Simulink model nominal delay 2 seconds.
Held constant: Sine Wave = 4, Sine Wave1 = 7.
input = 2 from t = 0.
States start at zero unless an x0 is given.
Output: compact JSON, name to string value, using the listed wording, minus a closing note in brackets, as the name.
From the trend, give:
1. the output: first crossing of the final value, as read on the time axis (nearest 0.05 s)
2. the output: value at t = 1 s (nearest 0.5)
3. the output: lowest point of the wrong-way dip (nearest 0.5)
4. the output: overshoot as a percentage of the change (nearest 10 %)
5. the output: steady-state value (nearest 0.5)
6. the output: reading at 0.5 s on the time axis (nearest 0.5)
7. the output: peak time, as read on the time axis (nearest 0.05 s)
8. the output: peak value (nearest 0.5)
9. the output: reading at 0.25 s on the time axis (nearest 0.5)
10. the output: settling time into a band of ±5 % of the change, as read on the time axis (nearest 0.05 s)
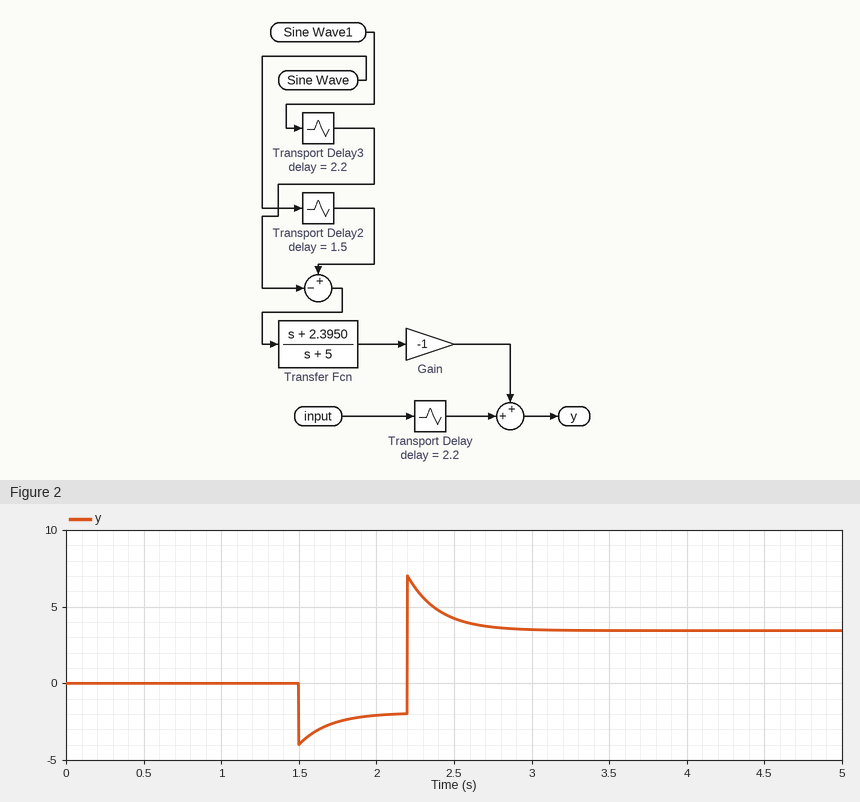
{"the output: first crossing of the final value, as read on the time axis": "2.20 s", "the output: value at t = 1 s": "0.0", "the output: lowest point of the wrong-way dip": "-4.0", "the output: overshoot as a percentage of the change": "100 %", "the output: steady-state value": "3.5", "the output: reading at 0.5 s on the time axis": "0.0", "the output: peak time, as read on the time axis": "2.20 s", "the output: peak value": "7.0", "the output: reading at 0.25 s on the time axis": "0.0", "the output: settling time into a band of ±5 % of the change, as read on the time axis": "2.80 s"}
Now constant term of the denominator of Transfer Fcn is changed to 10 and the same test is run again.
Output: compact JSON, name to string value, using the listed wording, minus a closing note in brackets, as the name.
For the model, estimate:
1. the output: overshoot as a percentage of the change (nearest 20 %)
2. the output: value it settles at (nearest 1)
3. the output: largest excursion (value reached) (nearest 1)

{"the output: overshoot as a percentage of the change": "200 %", "the output: value it settles at": "3", "the output: largest excursion (value reached)": "8"}
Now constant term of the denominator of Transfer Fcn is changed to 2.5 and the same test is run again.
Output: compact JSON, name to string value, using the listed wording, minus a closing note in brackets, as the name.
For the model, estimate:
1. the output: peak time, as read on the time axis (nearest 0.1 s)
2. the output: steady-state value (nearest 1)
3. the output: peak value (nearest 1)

{"the output: peak time, as read on the time axis": "2.2 s", "the output: steady-state value": "5", "the output: peak value": "5"}
